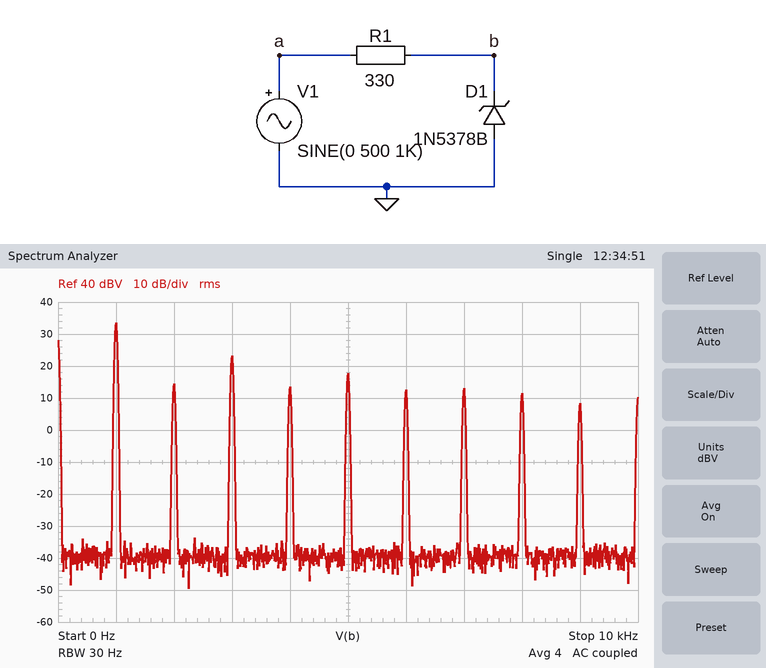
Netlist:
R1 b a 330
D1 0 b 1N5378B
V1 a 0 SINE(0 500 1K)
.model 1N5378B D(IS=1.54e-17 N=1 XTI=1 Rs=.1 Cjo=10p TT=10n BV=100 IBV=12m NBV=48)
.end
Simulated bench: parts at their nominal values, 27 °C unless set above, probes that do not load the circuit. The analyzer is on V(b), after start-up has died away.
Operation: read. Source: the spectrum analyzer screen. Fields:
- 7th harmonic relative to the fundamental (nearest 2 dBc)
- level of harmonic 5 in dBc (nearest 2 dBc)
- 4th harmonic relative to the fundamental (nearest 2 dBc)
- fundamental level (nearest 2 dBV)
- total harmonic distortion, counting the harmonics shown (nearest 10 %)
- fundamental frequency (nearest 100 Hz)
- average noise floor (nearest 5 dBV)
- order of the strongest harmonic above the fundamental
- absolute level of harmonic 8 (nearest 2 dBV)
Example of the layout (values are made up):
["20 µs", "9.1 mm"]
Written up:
["-20 dBc", "-16 dBc", "-20 dBc", "34 dBV", "40 %", "1.0 kHz", "-40 dBV", "3", "12 dBV"]
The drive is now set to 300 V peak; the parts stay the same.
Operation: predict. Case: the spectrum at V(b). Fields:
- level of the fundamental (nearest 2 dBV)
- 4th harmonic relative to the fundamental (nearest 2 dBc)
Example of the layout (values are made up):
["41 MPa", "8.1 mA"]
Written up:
["34 dBV", "-16 dBc"]
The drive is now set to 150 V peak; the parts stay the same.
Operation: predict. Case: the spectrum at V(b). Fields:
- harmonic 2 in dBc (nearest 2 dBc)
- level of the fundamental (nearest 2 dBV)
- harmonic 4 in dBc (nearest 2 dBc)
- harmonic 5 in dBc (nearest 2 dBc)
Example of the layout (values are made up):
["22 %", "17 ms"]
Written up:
["-10 dBc", "32 dBV", "-16 dBc", "-36 dBc"]
